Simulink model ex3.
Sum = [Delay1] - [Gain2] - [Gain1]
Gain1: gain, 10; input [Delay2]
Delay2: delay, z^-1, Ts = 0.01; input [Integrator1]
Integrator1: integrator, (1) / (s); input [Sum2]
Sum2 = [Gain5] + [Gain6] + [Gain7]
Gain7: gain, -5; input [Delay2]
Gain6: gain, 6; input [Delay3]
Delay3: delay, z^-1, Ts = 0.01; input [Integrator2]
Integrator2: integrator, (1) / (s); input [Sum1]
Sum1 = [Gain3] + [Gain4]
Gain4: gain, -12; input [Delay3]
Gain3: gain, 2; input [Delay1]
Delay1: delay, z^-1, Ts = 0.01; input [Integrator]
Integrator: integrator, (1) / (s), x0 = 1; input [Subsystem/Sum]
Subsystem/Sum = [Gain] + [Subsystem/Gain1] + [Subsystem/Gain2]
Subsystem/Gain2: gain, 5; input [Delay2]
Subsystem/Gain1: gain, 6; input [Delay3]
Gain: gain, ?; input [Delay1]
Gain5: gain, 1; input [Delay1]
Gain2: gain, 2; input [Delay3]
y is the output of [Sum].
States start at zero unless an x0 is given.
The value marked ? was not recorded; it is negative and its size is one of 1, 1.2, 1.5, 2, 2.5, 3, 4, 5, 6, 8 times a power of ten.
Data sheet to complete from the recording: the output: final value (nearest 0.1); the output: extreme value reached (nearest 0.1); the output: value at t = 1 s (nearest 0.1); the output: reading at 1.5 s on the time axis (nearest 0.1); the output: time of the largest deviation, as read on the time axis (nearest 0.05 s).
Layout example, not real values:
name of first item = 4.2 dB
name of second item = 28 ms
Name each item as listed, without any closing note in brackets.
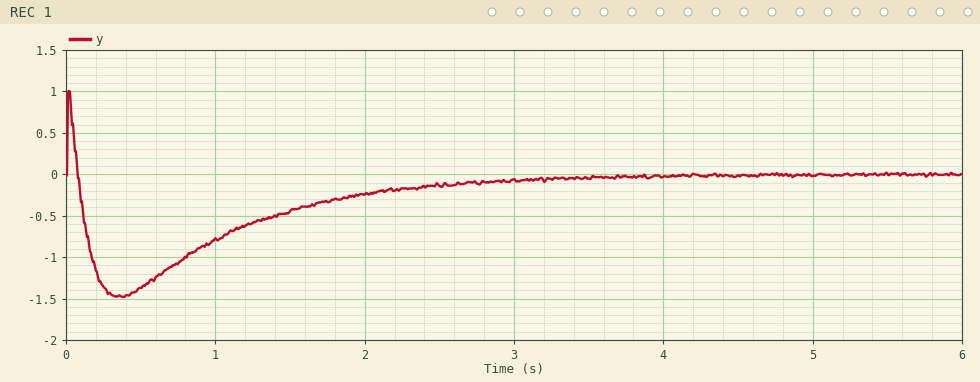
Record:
the output: final value = 0.0
the output: extreme value reached = -1.5
the output: value at t = 1 s = -0.8
the output: reading at 1.5 s on the time axis = -0.4
the output: time of the largest deviation, as read on the time axis = 0.35 s
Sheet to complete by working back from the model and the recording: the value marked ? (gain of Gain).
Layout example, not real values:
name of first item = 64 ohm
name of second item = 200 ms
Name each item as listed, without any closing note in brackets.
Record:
the value marked ? = -5
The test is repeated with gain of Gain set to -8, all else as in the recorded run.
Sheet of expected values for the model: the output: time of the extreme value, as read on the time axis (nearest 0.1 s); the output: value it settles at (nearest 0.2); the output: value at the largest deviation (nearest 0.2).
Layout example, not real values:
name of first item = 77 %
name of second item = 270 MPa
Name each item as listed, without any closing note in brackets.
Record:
the output: time of the extreme value, as read on the time axis = 0.3 s
the output: value it settles at = 0.0
the output: value at the largest deviation = -1.2
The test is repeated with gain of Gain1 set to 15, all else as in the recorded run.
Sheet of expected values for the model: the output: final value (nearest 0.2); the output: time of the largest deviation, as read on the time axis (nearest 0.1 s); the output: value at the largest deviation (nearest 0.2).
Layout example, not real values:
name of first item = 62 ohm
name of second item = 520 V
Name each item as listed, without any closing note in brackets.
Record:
the output: final value = 0.0
the output: time of the largest deviation, as read on the time axis = 0.3 s
the output: value at the largest deviation = -2.4
